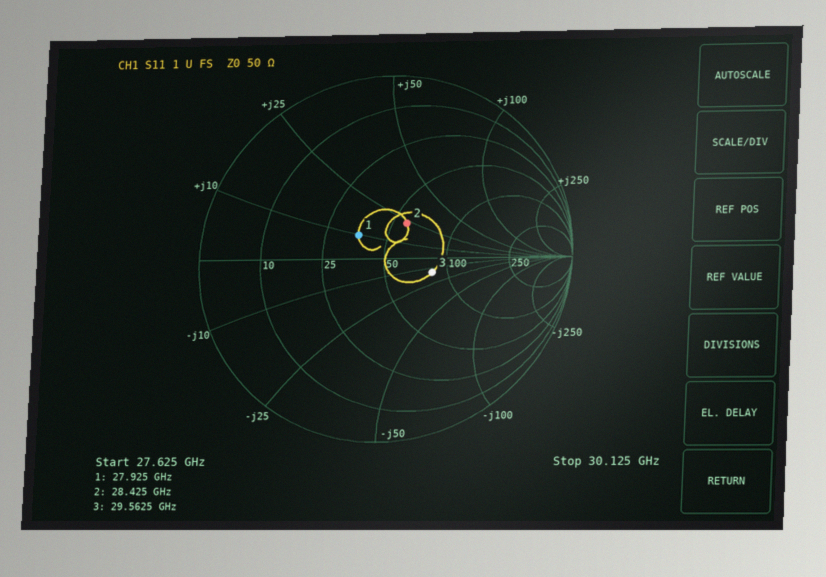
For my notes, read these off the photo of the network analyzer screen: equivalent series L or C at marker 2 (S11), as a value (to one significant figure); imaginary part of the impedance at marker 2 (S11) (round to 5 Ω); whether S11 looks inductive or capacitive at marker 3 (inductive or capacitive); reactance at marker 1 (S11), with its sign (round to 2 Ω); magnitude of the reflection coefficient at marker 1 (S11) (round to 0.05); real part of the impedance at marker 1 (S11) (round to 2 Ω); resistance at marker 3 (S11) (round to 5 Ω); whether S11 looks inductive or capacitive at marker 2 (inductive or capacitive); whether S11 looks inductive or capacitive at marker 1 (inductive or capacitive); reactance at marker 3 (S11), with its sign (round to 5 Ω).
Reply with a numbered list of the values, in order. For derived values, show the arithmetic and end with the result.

1. L = 25 Ω/(2π × 28.425 GHz) ≈ 140 pH, so 100 pH to one significant figure
2. +25 Ω
3. capacitive
4. +10 Ω
5. 0.20
6. 36 Ω
7. 85 Ω
8. inductive
9. inductive
10. -15 Ω
